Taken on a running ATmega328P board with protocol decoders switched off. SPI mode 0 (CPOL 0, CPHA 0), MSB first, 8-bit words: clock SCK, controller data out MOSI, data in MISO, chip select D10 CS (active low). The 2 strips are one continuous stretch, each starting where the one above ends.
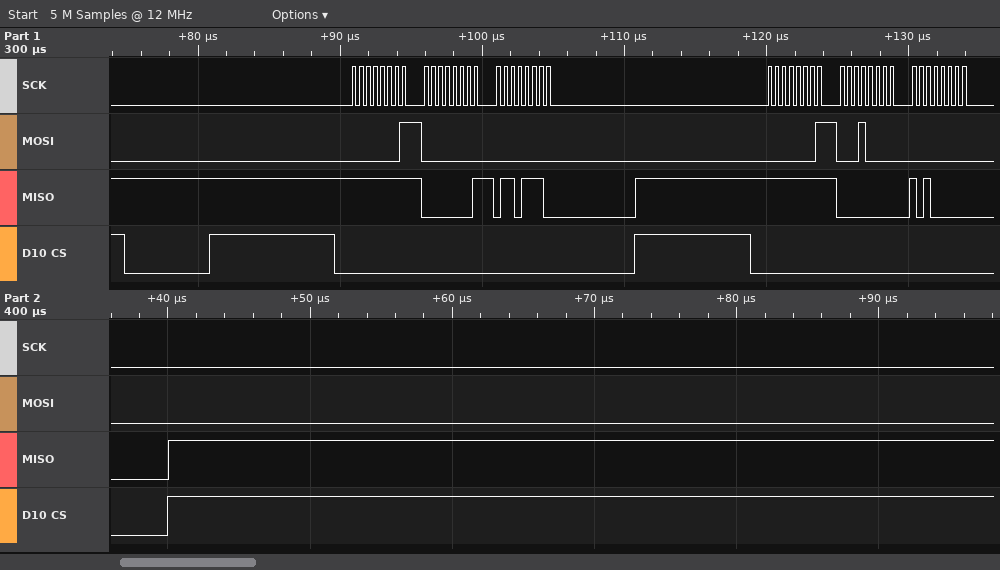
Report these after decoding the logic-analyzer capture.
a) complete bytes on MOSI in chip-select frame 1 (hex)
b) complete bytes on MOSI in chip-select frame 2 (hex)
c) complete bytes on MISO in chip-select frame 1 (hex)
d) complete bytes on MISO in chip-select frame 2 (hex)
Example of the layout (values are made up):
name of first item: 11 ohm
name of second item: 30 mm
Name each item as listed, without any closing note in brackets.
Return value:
complete bytes on MOSI in chip-select frame 1: 01 00 00
complete bytes on MOSI in chip-select frame 2: 01 10 00
complete bytes on MISO in chip-select frame 1: FF 01 6E
complete bytes on MISO in chip-select frame 2: FF 00 A0
